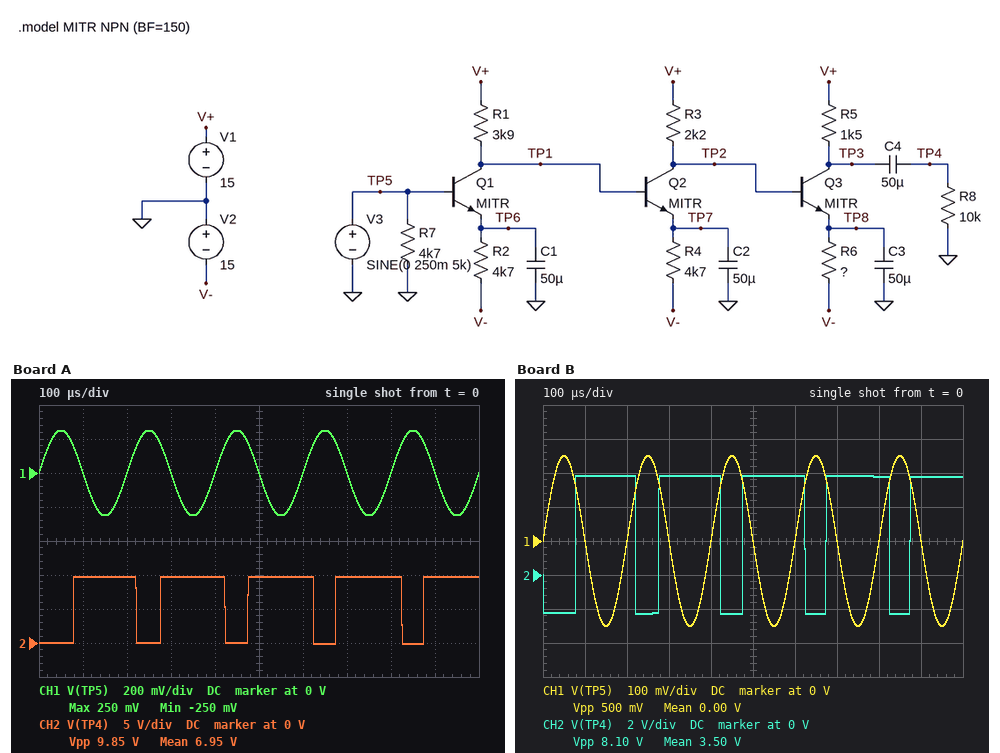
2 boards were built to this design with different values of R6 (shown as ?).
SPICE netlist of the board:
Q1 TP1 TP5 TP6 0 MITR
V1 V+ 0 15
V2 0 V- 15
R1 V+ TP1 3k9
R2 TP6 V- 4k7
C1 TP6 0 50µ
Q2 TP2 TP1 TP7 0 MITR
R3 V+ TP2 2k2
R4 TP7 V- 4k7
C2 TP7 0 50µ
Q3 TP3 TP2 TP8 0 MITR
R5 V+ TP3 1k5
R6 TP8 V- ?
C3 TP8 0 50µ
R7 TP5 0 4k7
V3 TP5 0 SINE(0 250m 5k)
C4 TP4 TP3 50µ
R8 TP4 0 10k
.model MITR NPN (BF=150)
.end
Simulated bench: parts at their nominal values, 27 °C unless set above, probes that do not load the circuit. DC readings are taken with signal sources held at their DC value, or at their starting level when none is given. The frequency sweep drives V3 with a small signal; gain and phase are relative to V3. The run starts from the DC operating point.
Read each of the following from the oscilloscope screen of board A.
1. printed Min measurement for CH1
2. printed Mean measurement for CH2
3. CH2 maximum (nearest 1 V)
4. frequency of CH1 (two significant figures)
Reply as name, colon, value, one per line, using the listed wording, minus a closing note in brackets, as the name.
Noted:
printed Min measurement for CH1: -250 mV
printed Mean measurement for CH2: 6.95 V
CH2 maximum: 10 V
frequency of CH1: 5.0 kHz
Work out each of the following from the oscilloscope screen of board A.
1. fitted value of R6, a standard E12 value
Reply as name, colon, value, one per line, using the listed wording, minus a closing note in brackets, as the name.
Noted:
fitted value of R6, a standard E12 value: 2.2 kΩ
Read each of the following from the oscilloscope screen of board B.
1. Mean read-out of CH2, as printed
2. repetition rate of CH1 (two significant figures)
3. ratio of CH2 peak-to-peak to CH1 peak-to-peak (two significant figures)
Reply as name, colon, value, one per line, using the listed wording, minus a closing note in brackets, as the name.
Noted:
Mean read-out of CH2, as printed: 3.50 V
repetition rate of CH1: 5.0 kHz
ratio of CH2 peak-to-peak to CH1 peak-to-peak: 16
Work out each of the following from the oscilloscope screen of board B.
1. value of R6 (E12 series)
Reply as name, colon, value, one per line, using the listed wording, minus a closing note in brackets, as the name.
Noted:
value of R6: 4.7 kΩ
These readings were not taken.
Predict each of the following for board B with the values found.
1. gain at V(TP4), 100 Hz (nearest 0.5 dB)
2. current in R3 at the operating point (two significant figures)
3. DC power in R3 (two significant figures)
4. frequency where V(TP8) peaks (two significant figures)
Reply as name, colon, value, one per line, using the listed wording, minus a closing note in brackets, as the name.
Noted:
gain at V(TP4), 100 Hz: 105.5 dB
current in R3 at the operating point: 3.7 mA
DC power in R3: 30 mW
frequency where V(TP8) peaks: 280 Hz
